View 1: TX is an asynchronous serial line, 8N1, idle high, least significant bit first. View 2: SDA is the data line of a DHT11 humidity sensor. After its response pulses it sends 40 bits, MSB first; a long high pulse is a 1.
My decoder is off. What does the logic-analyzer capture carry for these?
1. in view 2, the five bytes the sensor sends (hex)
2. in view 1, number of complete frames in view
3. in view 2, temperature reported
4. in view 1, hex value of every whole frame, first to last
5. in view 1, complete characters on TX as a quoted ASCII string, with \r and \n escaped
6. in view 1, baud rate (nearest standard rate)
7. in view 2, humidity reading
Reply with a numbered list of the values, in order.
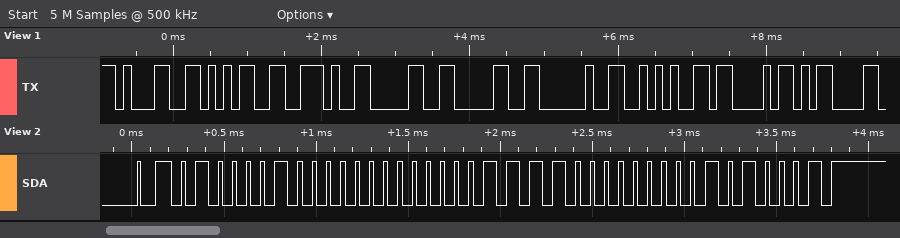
1. 42 00 0F 00 51
2. 9
3. 15.0 °C
4. 31 35 2E 30 30 20 2A 43 0D
5. "15.00 *C\r"
6. 9600 baud
7. 66 %
